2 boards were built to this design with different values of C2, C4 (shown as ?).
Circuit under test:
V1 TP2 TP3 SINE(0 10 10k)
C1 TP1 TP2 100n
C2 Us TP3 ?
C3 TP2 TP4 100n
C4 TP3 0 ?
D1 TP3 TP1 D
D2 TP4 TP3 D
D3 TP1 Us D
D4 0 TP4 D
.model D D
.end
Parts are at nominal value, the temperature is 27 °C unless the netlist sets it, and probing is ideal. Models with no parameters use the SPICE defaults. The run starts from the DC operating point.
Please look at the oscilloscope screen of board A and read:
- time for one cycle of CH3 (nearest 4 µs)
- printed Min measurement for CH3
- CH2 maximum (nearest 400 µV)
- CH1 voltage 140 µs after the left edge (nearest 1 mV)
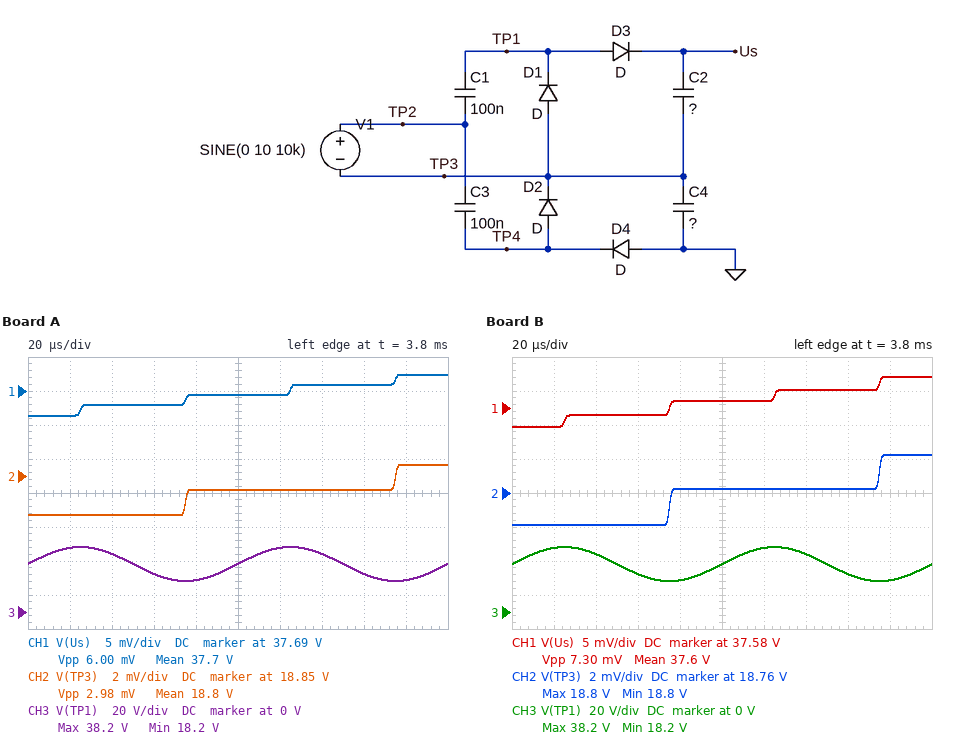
100 µs
18.2 V
18.8468 V
37.691 V
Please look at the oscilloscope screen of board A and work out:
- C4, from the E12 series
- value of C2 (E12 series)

47 nF
47 nF
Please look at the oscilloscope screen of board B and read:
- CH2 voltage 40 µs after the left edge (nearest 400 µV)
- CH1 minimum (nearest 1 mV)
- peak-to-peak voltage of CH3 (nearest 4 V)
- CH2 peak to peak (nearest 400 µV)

18.7600 V
37.577 V
20 V
4.0 mV
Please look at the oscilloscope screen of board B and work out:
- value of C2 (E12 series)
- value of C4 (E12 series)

82 nF
220 nF
